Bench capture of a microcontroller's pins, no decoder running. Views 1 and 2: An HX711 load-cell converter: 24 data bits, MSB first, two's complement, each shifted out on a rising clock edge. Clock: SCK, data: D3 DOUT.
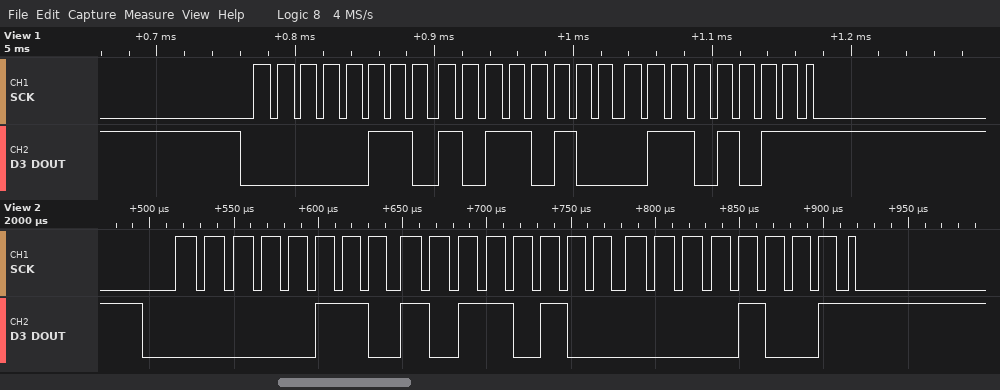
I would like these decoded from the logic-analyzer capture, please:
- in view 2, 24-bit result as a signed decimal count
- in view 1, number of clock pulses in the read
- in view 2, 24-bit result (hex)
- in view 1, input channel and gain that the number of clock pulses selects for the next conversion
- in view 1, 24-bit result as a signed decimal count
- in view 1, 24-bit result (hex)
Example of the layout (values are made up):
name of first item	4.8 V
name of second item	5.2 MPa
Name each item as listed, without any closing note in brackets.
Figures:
in view 2, 24-bit result as a signed decimal count	439305
in view 1, number of clock pulses in the read	25
in view 2, 24-bit result	0x06B409
in view 1, input channel and gain that the number of clock pulses selects for the next conversion	channel A, gain 128
in view 1, 24-bit result as a signed decimal count	439403
in view 1, 24-bit result	0x06B46B
